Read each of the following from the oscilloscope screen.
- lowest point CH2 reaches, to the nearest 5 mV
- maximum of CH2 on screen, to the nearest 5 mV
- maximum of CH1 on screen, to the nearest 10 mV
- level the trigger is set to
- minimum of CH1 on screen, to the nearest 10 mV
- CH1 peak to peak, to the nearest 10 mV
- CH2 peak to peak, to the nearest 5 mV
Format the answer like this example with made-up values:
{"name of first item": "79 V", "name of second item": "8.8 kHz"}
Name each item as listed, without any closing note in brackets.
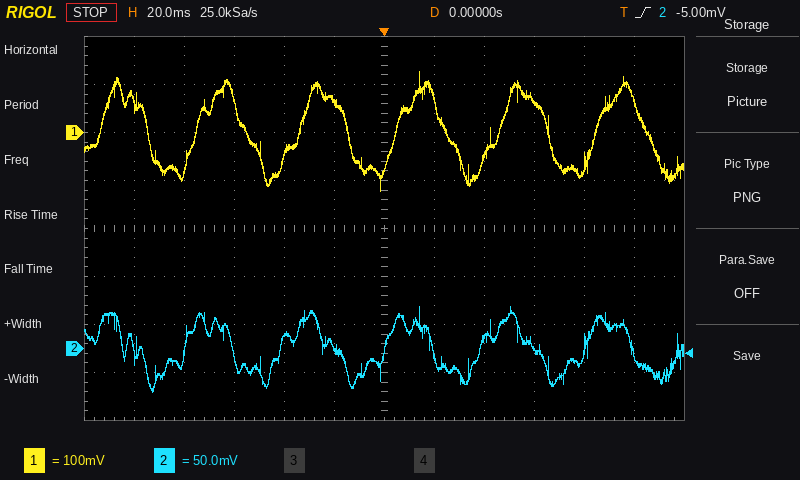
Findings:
{"lowest point CH2 reaches, to the nearest 5 mV": "-45 mV", "maximum of CH2 on screen, to the nearest 5 mV": "45 mV", "maximum of CH1 on screen, to the nearest 10 mV": "130 mV", "level the trigger is set to": "-5.00 mV", "minimum of CH1 on screen, to the nearest 10 mV": "-120 mV", "CH1 peak to peak, to the nearest 10 mV": "250 mV", "CH2 peak to peak, to the nearest 5 mV": "90 mV"}
